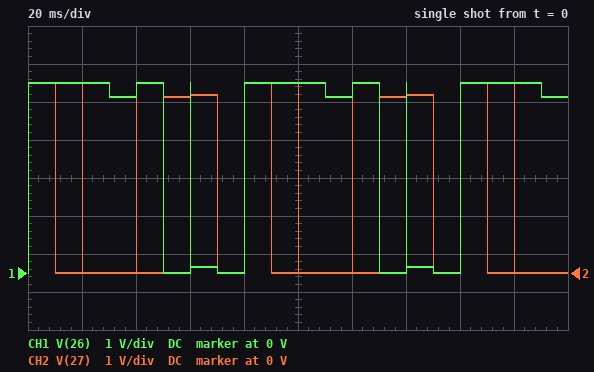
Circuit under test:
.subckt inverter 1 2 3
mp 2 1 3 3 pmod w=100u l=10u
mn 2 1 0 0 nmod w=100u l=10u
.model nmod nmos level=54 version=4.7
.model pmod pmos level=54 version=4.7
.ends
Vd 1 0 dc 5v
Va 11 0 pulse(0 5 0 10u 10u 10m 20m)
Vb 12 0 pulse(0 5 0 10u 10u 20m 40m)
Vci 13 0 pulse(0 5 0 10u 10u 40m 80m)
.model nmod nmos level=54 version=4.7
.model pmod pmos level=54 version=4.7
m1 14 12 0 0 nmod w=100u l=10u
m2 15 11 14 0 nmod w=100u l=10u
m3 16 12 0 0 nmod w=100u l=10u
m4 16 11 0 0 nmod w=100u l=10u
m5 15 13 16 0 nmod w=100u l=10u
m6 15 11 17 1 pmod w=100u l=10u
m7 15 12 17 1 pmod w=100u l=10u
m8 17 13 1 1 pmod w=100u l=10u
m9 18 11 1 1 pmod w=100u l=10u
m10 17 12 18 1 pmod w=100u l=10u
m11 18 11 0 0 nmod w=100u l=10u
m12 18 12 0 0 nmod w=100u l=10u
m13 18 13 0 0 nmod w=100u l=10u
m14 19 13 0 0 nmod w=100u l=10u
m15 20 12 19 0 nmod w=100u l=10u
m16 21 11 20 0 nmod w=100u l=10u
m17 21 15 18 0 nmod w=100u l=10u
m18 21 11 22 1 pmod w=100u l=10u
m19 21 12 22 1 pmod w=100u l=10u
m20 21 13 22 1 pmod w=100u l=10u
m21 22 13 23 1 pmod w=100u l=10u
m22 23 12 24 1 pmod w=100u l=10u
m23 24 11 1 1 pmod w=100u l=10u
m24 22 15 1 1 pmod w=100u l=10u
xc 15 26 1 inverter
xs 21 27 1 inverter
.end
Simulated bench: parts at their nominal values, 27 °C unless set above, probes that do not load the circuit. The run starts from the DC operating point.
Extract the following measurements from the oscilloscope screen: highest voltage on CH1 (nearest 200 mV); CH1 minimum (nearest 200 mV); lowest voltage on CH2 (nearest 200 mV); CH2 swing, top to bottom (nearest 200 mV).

5.0 V
0 V
0 V
5.0 V
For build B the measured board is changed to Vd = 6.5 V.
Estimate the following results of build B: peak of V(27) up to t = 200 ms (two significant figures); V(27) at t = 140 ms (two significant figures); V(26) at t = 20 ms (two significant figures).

6.3 V
5.1 V
6.5 V
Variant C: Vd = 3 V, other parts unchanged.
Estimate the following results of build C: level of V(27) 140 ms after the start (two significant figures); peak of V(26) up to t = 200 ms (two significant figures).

2.9 V
3.0 V
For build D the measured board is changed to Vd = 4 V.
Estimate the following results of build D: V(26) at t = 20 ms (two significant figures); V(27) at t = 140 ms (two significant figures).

4.0 V
3.8 V
